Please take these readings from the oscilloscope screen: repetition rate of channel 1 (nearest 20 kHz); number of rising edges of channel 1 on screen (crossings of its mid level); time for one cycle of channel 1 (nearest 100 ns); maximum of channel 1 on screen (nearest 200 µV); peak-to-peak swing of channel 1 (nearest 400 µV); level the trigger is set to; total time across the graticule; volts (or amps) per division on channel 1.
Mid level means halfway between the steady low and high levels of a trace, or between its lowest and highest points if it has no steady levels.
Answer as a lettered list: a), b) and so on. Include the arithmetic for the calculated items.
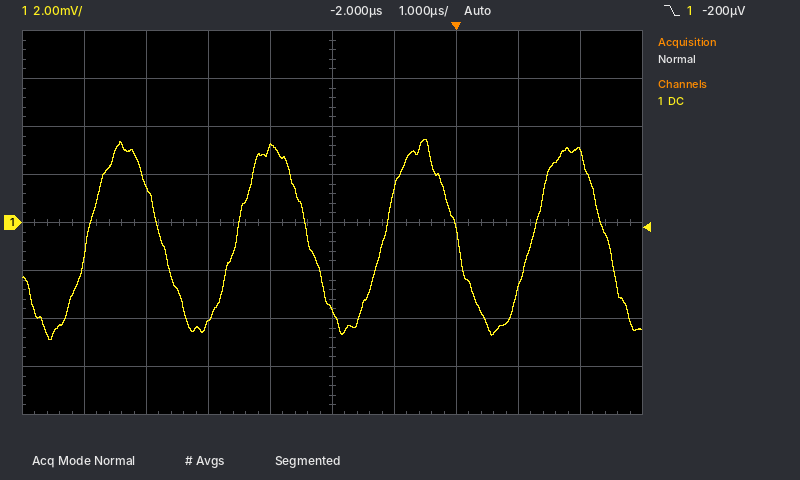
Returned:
a) 1 / 2.4 µs ≈ 417 kHz, so 420 kHz to the nearest 20 kHz
b) 4
c) 2.4 µs
d) 3.4 mV
e) 8.4 mV
f) -200 µV
g) 10 µs
h) 2 mV
